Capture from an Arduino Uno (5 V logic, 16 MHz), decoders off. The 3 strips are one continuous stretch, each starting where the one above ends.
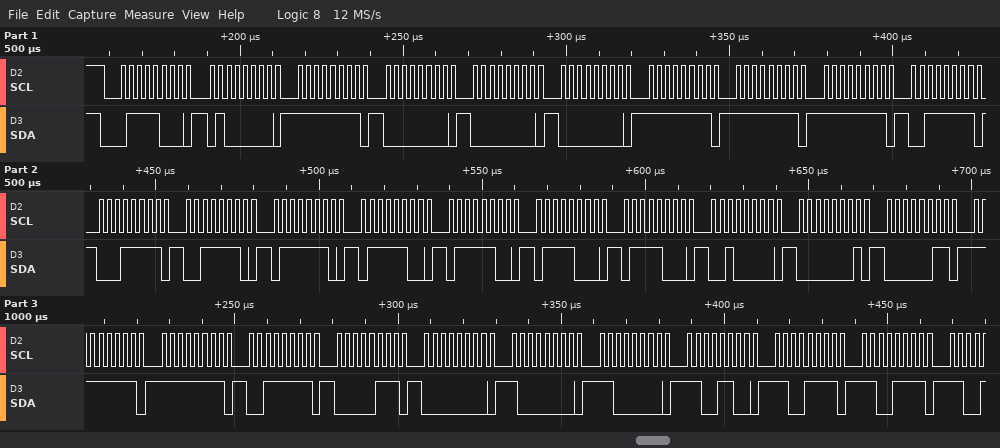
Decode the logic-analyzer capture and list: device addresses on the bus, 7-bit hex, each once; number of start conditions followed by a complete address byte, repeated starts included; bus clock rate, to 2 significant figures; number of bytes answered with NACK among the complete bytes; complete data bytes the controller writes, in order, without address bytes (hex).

0x3C
1
400 kHz
0
40 FF 00 00 00 FF FF FF 3F 1F 3E 7E 7C 7C 78 78 20 01 03 FF FF 3F 07 00 80 C0 CC CF CF
